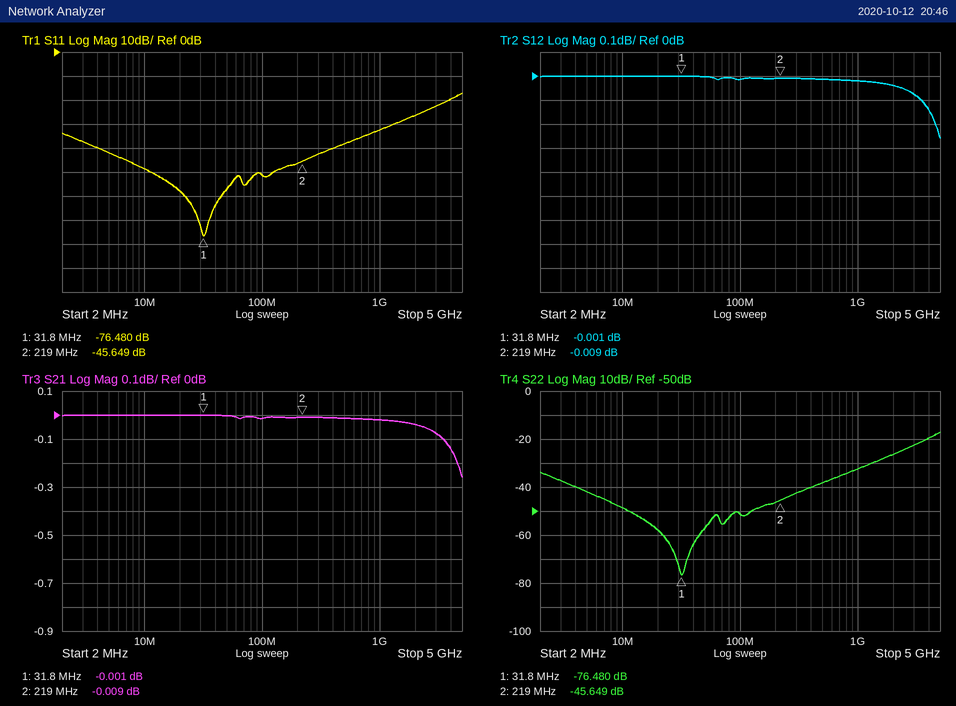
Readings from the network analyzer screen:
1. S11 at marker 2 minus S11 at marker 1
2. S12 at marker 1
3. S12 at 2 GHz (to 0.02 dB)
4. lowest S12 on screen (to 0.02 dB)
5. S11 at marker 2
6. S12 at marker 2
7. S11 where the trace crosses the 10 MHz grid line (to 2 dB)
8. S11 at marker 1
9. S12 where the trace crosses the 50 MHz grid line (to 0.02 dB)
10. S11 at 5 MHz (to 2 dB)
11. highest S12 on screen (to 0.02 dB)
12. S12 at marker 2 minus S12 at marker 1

30.831 dB
-0.001 dB
-0.04 dB
-0.26 dB
-45.649 dB
-0.009 dB
-48 dB
-76.480 dB
0.00 dB
-42 dB
0.00 dB
-0.008 dB
